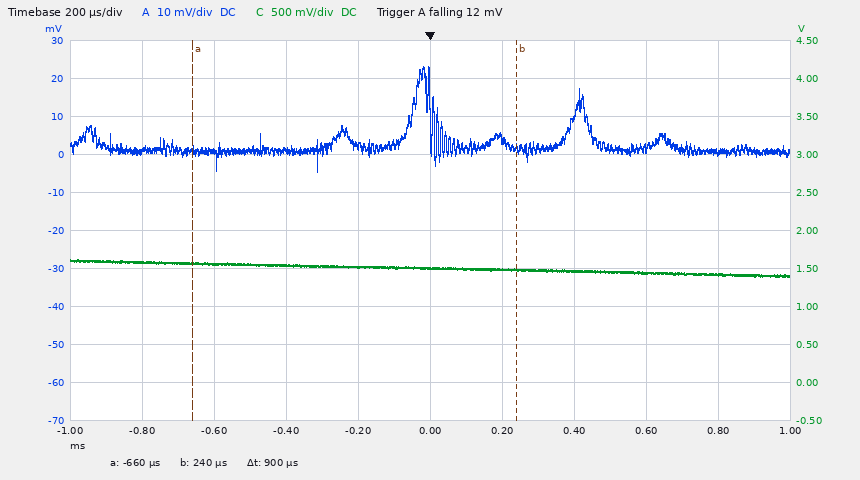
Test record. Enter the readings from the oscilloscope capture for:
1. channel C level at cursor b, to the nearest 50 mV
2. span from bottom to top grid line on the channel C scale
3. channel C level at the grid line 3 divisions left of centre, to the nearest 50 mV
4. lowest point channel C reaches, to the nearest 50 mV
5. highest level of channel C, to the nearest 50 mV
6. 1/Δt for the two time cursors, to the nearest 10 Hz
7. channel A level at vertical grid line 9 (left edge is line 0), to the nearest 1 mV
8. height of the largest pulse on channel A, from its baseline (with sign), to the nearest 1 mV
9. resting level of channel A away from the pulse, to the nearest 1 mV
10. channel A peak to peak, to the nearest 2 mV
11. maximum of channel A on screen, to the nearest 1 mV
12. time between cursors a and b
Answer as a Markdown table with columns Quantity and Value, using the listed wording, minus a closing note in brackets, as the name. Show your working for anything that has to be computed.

| Quantity | Value |
|---|---|
| channel C level at cursor b, to the nearest 50 mV | 1.50 V |
| span from bottom to top grid line on the channel C scale | 5 V |
| channel C level at the grid line 3 divisions left of centre, to the nearest 50 mV | 1.55 V |
| lowest point channel C reaches, to the nearest 50 mV | 1.40 V |
| highest level of channel C, to the nearest 50 mV | 1.60 V |
| 1/Δt for the two time cursors, to the nearest 10 Hz | 1 / 900 µs ≈ 1.11 kHz |
| channel A level at vertical grid line 9 (left edge is line 0), to the nearest 1 mV | 1 mV |
| height of the largest pulse on channel A, from its baseline (with sign), to the nearest 1 mV | 23 mV − (1 mV) = +22 mV |
| resting level of channel A away from the pulse, to the nearest 1 mV | 1 mV |
| channel A peak to peak, to the nearest 2 mV | 28 mV |
| maximum of channel A on screen, to the nearest 1 mV | 23 mV |
| time between cursors a and b | 900 µs |
